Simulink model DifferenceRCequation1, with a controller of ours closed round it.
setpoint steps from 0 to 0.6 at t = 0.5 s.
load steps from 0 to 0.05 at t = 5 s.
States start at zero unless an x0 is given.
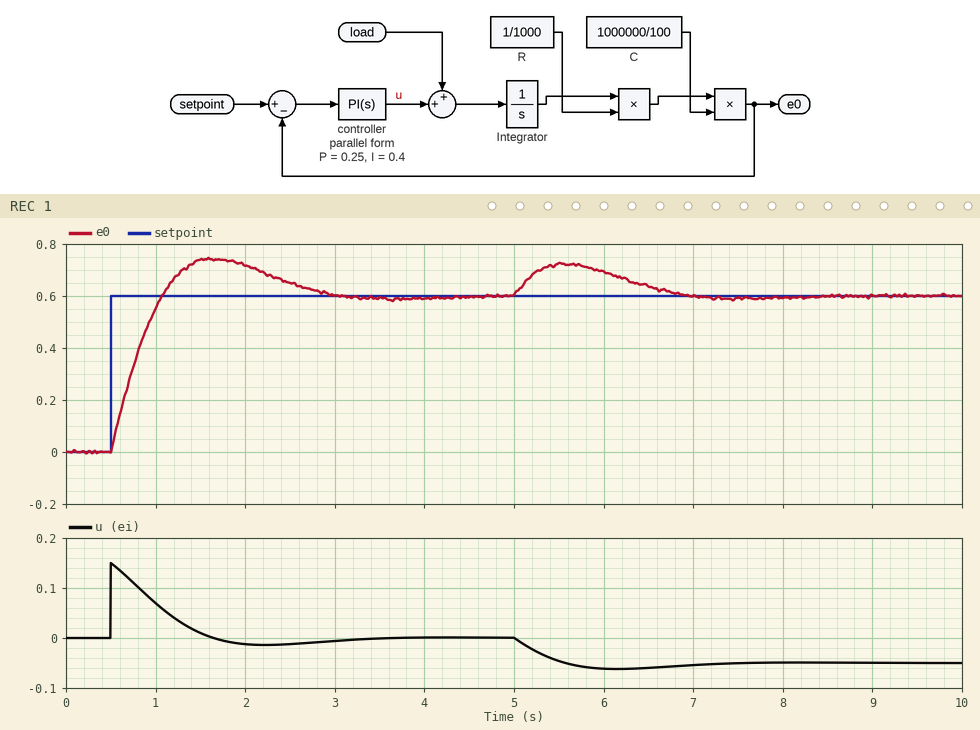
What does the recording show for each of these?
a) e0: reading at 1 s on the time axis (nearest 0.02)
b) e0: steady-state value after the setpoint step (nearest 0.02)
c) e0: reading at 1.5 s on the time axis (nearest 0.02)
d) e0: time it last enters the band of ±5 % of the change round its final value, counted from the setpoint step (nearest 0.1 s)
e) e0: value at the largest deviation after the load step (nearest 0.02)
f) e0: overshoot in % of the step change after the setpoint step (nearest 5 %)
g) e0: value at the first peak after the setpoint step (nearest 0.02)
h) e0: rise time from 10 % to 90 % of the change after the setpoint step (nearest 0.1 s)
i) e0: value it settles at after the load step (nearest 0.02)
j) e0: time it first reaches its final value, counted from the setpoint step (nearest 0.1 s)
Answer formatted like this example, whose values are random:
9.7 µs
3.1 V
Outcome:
0.56
0.60
0.74
2.2 s
0.72
25 %
0.74
0.4 s
0.60
0.6 s
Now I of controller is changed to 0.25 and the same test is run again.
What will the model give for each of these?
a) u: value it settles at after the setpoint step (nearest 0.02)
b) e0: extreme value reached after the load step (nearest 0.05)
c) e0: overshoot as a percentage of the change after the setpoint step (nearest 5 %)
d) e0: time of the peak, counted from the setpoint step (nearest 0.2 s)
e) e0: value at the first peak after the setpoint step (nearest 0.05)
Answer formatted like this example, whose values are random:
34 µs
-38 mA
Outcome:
0.00
0.75
20 %
1.4 s
0.70
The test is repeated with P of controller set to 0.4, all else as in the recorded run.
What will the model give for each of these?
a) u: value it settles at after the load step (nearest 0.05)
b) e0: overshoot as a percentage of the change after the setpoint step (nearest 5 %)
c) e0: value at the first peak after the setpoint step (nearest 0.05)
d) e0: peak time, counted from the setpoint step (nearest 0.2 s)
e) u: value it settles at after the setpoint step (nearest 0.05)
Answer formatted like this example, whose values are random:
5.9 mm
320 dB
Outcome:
-0.05
15 %
0.70
1.0 s
0.00
